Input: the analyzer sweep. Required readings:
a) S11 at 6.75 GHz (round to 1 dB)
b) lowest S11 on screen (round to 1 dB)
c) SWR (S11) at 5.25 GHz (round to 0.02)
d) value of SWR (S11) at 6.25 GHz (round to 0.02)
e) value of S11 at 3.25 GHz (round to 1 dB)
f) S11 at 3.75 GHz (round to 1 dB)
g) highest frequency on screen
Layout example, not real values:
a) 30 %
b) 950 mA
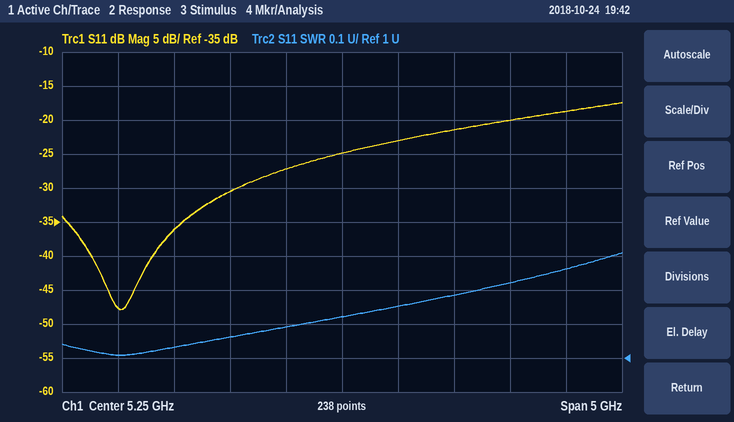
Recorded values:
a) -20 dB
b) -48 dB
c) 1.12
d) 1.18
e) -48 dB
f) -36 dB
g) 7.75 GHz
